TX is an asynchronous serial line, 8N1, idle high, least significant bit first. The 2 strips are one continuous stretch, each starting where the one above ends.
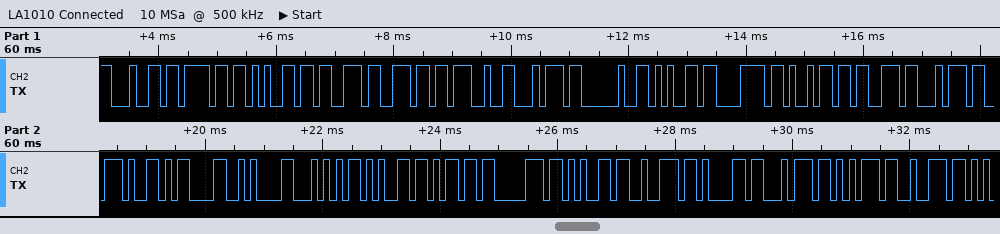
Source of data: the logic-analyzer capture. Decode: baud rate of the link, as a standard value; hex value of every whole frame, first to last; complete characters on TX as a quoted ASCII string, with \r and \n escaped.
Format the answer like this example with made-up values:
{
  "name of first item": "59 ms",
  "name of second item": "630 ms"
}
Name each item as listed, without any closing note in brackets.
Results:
{
  "baud rate of the link, as a standard value": "9600 baud",
  "hex value of every whole frame, first to last": "0x64 0x6F 0x65 0x73 0x6E 0x27 0x74 0x20 0x65 0x78 0x69 0x73 0x74 0x2E 0x0D 0x0A 0x54 0x65 0x6D 0x70 0x65 0x72 0x61 0x74 0x75 0x72",
  "complete characters on TX as a quoted ASCII string, with \\r and \\n escaped": "\"doesn't exist.\\r\\nTemperatur\""
}
